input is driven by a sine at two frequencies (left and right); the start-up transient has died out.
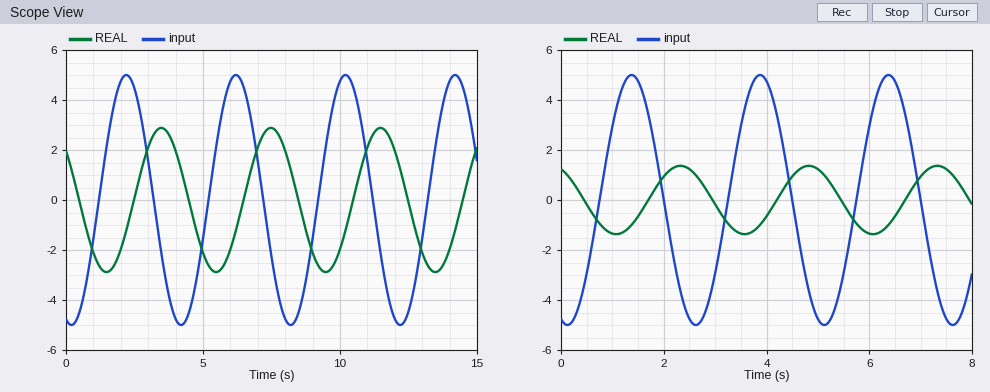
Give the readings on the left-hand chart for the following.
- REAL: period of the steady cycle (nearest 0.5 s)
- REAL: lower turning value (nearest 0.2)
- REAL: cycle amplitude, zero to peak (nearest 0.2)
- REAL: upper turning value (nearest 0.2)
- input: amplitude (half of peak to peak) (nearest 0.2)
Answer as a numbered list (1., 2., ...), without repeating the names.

1. 4.0 s
2. -2.8
3. 2.8
4. 2.8
5. 5.0
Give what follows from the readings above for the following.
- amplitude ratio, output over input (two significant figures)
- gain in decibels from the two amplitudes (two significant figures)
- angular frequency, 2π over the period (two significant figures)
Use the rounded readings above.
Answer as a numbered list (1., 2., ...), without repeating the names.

1. 0.56
2. -5.0 dB
3. 1.6 rad/s
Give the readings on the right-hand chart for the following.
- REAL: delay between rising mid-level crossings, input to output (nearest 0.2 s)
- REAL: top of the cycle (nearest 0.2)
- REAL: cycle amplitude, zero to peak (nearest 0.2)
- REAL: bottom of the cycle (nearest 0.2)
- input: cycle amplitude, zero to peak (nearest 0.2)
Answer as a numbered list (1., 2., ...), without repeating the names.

1. 1.0 s
2. 1.4
3. 1.4
4. -1.4
5. 5.0
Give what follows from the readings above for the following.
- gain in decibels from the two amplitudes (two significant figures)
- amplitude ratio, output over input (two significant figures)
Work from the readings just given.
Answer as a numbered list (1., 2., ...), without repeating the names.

1. -11 dB
2. 0.28
